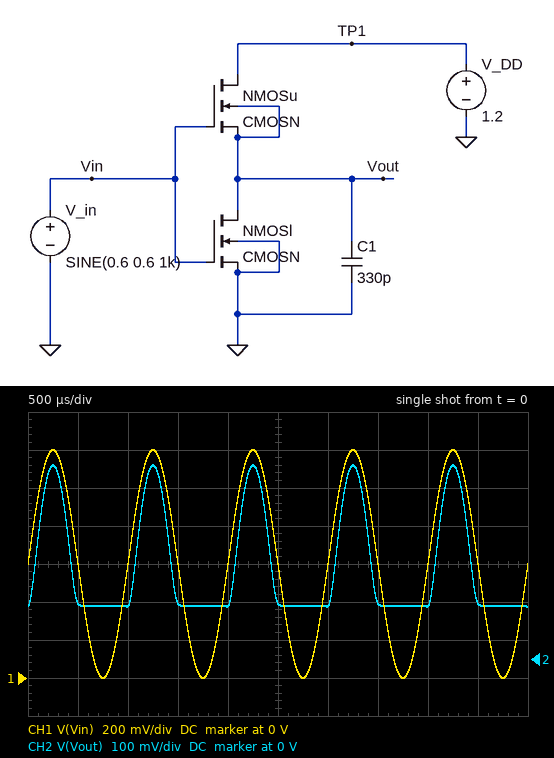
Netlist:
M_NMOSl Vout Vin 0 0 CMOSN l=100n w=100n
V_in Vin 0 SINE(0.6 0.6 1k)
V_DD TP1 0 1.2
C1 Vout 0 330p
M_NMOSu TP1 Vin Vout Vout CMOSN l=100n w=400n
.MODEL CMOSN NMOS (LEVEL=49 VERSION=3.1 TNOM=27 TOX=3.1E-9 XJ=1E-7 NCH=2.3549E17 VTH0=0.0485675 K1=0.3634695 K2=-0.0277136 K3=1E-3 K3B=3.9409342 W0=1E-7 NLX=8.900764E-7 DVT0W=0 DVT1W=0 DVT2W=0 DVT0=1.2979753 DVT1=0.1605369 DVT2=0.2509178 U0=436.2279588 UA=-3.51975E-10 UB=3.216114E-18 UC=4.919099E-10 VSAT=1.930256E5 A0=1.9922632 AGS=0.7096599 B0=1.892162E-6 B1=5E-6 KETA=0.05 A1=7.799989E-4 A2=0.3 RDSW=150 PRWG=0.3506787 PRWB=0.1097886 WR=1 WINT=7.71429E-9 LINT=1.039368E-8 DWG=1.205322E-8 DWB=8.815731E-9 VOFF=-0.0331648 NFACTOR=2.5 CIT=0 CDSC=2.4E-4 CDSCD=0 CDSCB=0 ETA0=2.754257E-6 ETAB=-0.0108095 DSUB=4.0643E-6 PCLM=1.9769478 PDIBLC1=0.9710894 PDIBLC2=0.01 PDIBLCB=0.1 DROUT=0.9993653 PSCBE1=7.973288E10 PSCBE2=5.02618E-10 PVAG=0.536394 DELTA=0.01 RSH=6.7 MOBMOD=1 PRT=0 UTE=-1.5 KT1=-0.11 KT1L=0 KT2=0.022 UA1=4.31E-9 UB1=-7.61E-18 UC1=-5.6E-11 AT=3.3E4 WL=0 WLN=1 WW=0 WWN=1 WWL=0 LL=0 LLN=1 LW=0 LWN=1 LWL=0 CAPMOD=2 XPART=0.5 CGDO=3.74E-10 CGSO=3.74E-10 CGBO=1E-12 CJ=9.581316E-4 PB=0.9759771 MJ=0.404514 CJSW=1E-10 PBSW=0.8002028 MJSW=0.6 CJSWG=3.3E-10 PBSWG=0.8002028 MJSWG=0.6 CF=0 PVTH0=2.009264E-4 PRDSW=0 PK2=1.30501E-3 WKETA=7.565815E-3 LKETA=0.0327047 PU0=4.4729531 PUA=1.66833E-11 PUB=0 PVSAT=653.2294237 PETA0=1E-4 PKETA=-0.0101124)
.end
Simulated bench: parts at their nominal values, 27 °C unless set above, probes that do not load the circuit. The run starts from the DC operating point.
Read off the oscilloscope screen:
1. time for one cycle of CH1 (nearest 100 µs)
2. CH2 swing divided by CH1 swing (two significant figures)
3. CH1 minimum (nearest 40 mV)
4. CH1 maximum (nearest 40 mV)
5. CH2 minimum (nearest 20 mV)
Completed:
1.0 ms
0.31
0 V
1.20 V
140 mV
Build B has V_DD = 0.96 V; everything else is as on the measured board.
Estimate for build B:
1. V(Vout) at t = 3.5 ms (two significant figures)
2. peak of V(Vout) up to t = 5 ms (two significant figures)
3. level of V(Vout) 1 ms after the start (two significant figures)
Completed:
140 mV
490 mV
130 mV
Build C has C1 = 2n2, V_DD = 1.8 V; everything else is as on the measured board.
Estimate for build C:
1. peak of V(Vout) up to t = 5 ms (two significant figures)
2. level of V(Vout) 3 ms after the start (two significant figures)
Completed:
550 mV
190 mV
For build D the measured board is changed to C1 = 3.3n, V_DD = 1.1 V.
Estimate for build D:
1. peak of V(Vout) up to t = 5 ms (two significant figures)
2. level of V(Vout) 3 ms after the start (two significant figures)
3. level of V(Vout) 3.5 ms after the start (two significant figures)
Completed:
500 mV
180 mV
190 mV
